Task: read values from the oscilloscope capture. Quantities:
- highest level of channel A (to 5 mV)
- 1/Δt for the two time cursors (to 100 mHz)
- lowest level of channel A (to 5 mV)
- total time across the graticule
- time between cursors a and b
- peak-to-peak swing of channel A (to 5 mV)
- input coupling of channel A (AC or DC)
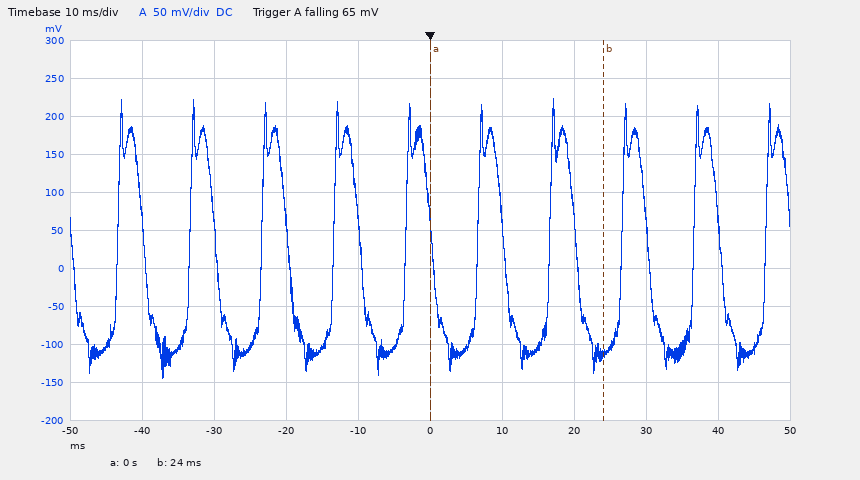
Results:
225 mV
41.7 Hz
-145 mV
100 ms
24 ms
370 mV
DC
